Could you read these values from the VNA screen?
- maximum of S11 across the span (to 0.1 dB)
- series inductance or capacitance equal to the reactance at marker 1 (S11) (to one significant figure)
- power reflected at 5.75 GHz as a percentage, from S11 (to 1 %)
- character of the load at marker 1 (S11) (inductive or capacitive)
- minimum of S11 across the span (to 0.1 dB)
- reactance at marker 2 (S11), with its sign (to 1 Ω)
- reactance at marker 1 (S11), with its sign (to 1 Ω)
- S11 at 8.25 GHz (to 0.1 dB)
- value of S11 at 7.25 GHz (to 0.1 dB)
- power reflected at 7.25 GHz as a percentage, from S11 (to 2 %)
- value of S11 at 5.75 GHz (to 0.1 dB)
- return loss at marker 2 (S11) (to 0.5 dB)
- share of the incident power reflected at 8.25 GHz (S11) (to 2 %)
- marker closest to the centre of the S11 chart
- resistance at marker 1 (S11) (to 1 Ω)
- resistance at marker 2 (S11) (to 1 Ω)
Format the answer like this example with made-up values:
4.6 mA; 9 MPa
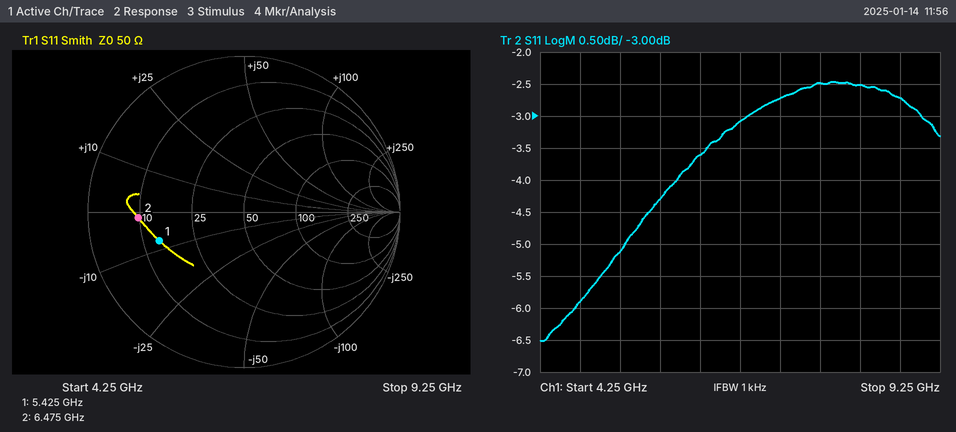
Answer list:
-2.5 dB; 4 pF; 37 %; capacitive; -6.5 dB; -1 Ω; -8 Ω; -2.5 dB; -2.7 dB; 54 %; -4.3 dB; 3.5 dB; 56 %; marker 1; 14 Ω; 10 Ω
